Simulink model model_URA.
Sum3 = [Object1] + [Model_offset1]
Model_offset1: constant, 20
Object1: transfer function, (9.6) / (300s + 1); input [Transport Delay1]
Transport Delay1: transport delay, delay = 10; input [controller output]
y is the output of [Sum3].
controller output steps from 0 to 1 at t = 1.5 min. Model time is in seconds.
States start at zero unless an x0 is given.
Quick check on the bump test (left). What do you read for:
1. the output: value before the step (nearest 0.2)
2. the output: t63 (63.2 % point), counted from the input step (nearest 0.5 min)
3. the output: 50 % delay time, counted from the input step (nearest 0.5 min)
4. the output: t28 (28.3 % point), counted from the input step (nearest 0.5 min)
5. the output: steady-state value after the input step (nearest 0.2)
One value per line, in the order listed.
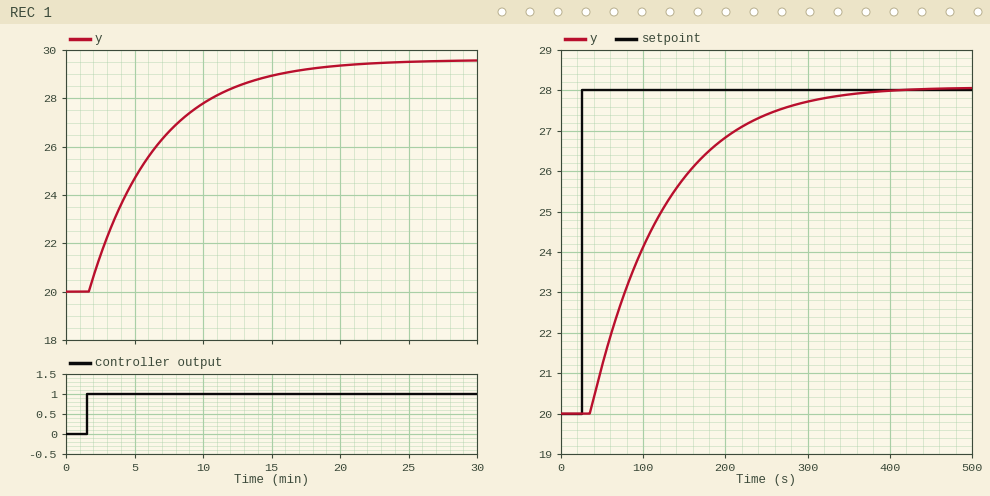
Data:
20.0
5.0 min
3.5 min
2.0 min
29.6
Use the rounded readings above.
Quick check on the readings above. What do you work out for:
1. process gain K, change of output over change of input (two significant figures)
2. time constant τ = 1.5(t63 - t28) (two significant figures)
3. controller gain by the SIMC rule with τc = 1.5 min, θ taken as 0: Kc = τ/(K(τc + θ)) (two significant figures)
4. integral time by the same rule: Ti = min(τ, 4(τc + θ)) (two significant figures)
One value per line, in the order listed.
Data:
9.6
4.5 min
0.31
4.5 min
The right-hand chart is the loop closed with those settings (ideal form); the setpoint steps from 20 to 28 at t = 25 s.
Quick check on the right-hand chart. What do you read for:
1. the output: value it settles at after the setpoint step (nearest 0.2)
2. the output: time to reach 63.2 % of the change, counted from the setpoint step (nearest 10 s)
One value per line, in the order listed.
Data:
28.0
100 s
